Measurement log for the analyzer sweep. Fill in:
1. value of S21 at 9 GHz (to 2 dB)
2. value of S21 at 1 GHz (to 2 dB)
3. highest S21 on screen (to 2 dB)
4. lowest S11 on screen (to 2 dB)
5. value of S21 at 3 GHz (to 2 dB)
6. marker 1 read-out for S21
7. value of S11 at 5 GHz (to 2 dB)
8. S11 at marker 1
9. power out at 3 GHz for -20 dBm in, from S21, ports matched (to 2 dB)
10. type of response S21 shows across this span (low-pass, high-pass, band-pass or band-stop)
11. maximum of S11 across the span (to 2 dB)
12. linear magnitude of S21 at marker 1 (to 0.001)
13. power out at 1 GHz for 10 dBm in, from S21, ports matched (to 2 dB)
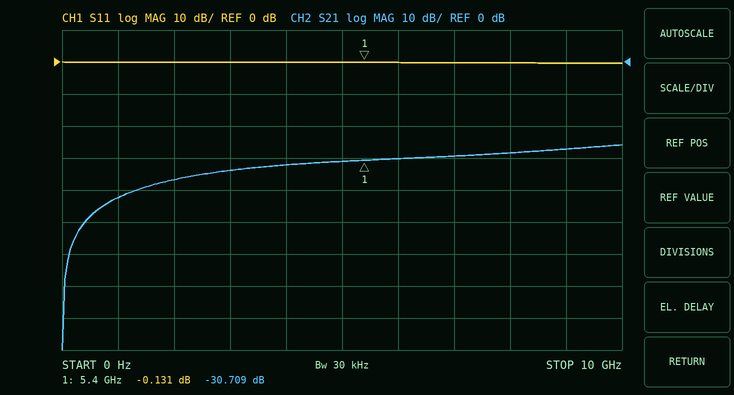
-28 dB
-42 dB
-26 dB
0 dB
-34 dB
-30.709 dB
0 dB
-0.131 dB
-54 dBm
high-pass
0 dB
0.029
-32 dBm
